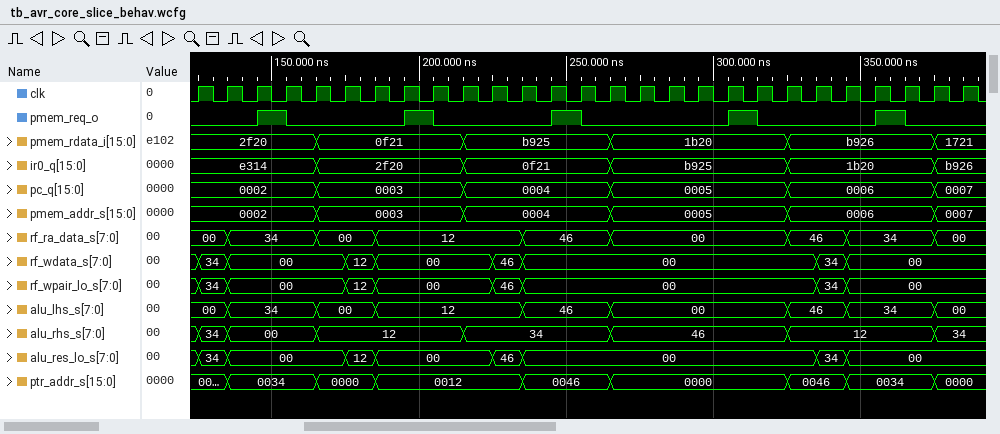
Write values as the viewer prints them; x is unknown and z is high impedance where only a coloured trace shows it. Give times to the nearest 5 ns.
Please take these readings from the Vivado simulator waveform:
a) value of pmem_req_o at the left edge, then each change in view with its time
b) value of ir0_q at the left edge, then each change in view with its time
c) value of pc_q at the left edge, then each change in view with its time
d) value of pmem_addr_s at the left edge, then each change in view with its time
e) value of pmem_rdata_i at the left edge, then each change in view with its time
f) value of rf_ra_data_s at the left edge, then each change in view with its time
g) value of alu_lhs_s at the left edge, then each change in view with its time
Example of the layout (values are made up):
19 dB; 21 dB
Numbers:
0, 1 at 145 ns, 0 at 155 ns, 1 at 195 ns, 0 at 205 ns, 1 at 245 ns, 0 at 255 ns, 1 at 305 ns, 0 at 315 ns, 1 at 355 ns, 0 at 365 ns; e314, 2f20 at 165 ns, 0f21 at 215 ns, b925 at 265 ns, 1b20 at 325 ns, b926 at 375 ns; 0002, 0003 at 165 ns, 0004 at 215 ns, 0005 at 265 ns, 0006 at 325 ns, 0007 at 375 ns; 0002, 0003 at 165 ns, 0004 at 215 ns, 0005 at 265 ns, 0006 at 325 ns, 0007 at 375 ns; 2f20, 0f21 at 165 ns, b925 at 215 ns, 1b20 at 265 ns, b926 at 325 ns, 1721 at 375 ns; 00, 34 at 135 ns, 00 at 165 ns, 12 at 185 ns, 46 at 235 ns, 00 at 265 ns, 46 at 325 ns, 34 at 345 ns, 00 at 375 ns; 00, 34 at 135 ns, 00 at 165 ns, 12 at 185 ns, 46 at 235 ns, 00 at 265 ns, 46 at 325 ns, 34 at 345 ns, 00 at 375 ns
